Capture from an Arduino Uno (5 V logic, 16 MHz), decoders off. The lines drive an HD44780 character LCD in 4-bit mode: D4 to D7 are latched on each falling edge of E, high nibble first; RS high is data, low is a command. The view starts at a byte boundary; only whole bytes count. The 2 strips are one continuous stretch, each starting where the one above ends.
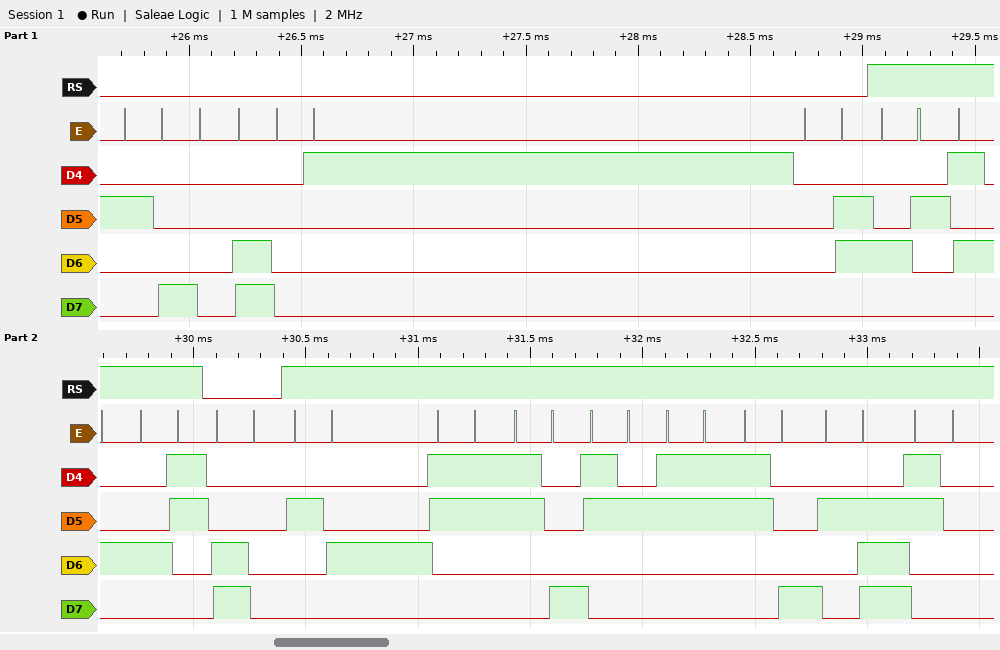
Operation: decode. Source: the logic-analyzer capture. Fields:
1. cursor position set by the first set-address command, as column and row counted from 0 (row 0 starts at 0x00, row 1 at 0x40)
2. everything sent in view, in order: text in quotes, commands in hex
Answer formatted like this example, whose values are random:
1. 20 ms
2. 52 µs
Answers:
1. column 0, row 1
2. 0x28 0x0C 0x01 0x06 "BTC" 0xC0 "$38238.0"
